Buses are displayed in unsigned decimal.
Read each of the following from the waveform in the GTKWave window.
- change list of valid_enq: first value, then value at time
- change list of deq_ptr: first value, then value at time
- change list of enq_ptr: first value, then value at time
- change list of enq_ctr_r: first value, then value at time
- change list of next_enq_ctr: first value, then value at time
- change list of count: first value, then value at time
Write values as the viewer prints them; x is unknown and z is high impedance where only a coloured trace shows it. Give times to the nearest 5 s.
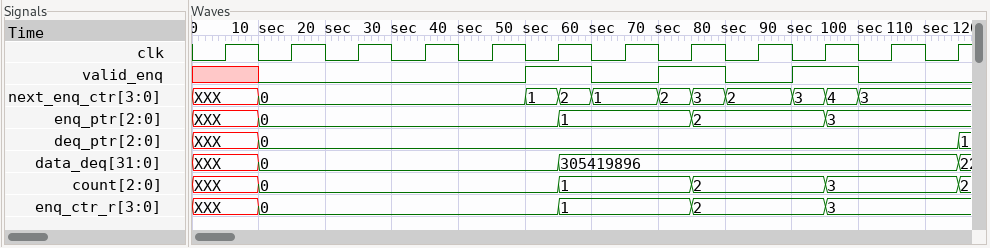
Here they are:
x, 0 at 10 s, 1 at 50 s, 0 at 60 s, 1 at 70 s, 0 at 80 s, 1 at 90 s, 0 at 100 s
XXX, 0 at 10 s, 1 at 115 s
XXX, 0 at 10 s, 1 at 55 s, 2 at 75 s, 3 at 95 s
XXX, 0 at 10 s, 1 at 55 s, 2 at 75 s, 3 at 95 s
XXX, 0 at 10 s, 1 at 50 s, 2 at 55 s, 1 at 60 s, 2 at 70 s, 3 at 75 s, 2 at 80 s, 3 at 90 s, 4 at 95 s, 3 at 100 s
XXX, 0 at 10 s, 1 at 55 s, 2 at 75 s, 3 at 95 s, 2 at 115 s
